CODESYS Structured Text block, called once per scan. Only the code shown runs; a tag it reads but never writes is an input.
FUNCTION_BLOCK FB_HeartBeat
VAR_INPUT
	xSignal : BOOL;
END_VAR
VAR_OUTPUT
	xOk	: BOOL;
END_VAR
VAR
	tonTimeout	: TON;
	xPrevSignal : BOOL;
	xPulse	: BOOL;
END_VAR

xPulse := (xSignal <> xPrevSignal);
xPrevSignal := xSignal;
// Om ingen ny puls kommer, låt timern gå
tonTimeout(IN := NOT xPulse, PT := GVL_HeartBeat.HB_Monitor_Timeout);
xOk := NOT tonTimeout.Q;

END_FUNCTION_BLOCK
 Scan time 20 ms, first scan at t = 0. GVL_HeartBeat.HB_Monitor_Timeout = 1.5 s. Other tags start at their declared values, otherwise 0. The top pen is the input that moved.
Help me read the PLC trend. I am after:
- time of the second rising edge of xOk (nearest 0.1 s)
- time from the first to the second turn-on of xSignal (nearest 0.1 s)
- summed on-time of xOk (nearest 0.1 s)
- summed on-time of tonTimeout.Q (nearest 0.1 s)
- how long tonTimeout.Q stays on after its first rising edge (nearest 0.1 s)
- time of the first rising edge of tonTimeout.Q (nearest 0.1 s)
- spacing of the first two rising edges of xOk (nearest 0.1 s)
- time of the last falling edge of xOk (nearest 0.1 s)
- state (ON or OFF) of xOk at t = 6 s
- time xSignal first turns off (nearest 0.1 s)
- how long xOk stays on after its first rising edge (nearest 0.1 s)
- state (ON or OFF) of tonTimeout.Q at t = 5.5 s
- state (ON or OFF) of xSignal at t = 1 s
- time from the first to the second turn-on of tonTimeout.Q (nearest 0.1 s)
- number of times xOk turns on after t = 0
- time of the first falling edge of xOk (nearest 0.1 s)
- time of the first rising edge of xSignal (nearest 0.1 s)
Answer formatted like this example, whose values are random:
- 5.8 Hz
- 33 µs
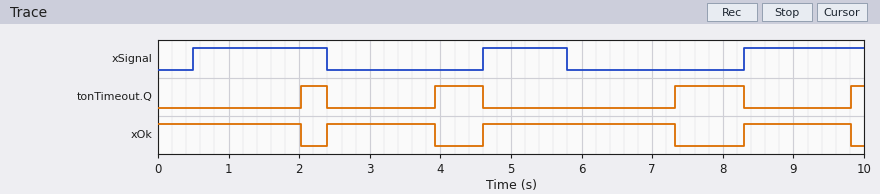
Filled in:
- 4.6 s
- 4.1 s
- 7.8 s
- 2.2 s
- 0.4 s
- 2.0 s
- 2.2 s
- 9.8 s
- ON
- 2.4 s
- 1.5 s
- OFF
- ON
- 1.9 s
- 3
- 2.0 s
- 0.5 s
